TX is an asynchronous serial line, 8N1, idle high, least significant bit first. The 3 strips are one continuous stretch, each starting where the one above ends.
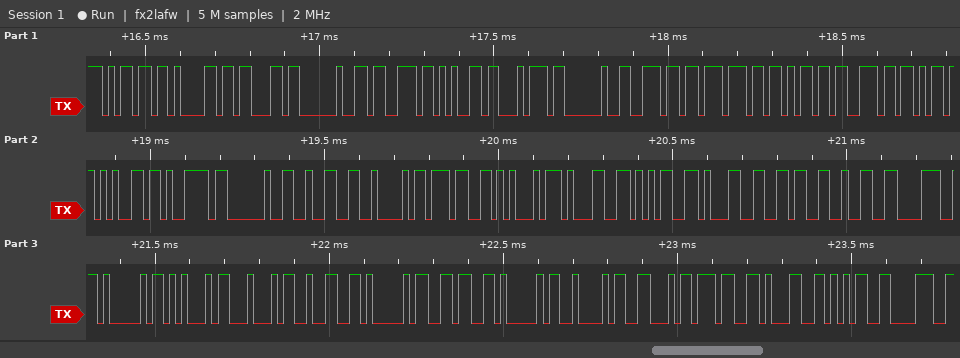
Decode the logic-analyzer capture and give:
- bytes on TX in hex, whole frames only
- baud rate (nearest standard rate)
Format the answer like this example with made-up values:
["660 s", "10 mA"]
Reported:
["6D 61 63 20 73 65 74 20 6E 77 6B 73 6B 65 79 20 32 42 37 45 31 35 31 36 32 38 41 45 44 32 41 36 41 42 46 37 31 35 38", "57600 baud"]
